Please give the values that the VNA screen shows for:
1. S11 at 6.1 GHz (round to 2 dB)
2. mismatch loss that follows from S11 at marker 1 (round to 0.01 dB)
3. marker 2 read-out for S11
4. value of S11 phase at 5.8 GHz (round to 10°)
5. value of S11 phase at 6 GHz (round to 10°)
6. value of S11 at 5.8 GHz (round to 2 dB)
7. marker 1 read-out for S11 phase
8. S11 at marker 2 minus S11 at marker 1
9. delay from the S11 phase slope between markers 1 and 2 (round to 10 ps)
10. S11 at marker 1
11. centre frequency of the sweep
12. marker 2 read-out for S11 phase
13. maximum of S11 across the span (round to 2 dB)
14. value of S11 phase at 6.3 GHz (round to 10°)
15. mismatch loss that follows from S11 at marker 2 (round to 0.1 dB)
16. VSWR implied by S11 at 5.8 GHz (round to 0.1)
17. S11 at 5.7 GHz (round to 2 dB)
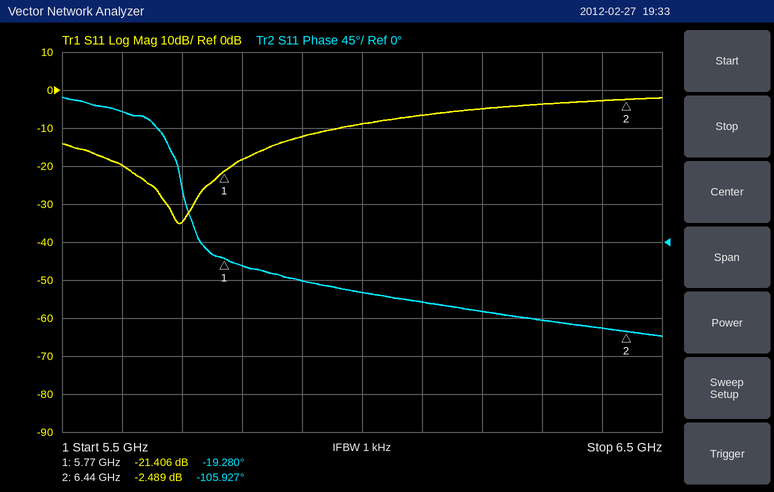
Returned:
-6 dB
0.03 dB
-2.489 dB
-30°
-60°
-18 dB
-19.280°
18.917 dB
360 ps
-21.406 dB
6 GHz
-105.927°
-2 dB
-90°
3.6 dB
1.3
-34 dB
